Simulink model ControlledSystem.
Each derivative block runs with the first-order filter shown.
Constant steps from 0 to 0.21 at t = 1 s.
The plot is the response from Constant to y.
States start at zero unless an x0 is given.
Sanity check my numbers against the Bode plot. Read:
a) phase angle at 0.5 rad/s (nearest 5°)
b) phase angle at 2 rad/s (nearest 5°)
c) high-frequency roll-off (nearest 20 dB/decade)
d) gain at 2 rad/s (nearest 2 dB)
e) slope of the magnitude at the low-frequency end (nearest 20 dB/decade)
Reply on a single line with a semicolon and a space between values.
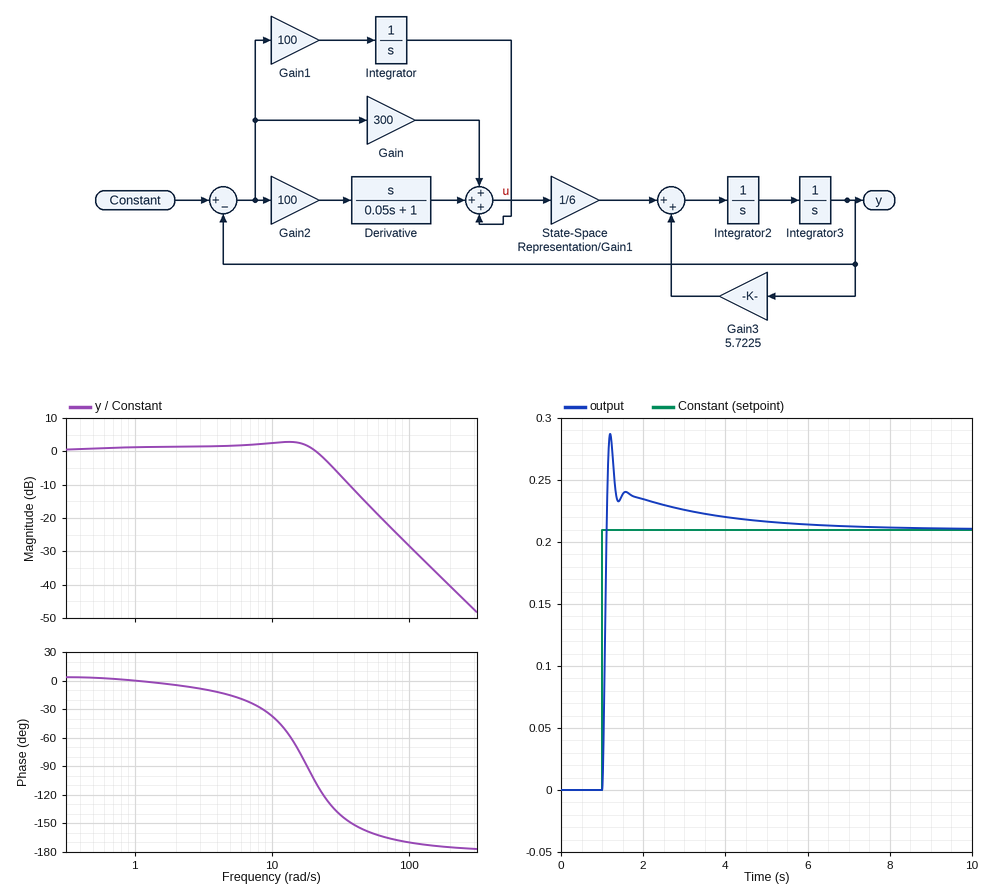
5°; -5°; -40 dB/decade; 2 dB; 0 dB/decade
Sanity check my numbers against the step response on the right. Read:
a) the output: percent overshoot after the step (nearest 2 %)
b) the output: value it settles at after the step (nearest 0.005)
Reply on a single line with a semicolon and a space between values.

36 %; 0.210
